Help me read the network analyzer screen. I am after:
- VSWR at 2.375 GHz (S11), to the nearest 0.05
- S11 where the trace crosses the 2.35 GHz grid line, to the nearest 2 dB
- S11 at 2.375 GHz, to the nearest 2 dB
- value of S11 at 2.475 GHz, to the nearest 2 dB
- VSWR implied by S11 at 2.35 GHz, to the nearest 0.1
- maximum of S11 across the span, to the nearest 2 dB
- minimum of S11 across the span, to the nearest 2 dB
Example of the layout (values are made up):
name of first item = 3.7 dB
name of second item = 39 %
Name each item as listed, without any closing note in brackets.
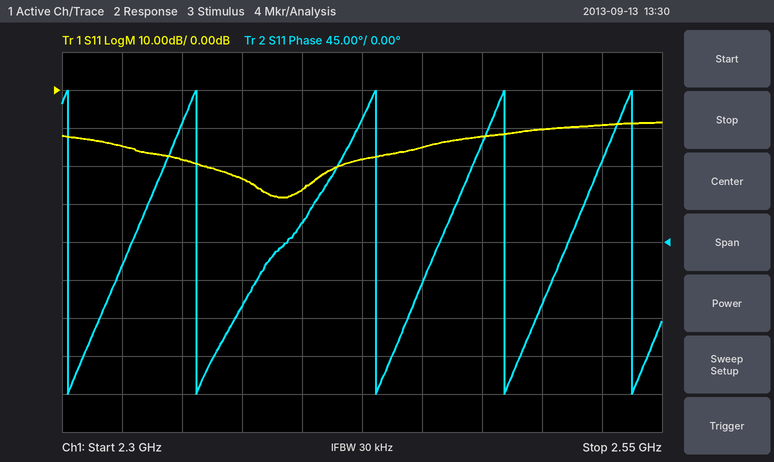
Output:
VSWR at 2.375 GHz (S11), to the nearest 0.05 = 1.15
S11 where the trace crosses the 2.35 GHz grid line, to the nearest 2 dB = -18 dB
S11 at 2.375 GHz, to the nearest 2 dB = -24 dB
value of S11 at 2.475 GHz, to the nearest 2 dB = -12 dB
VSWR implied by S11 at 2.35 GHz, to the nearest 0.1 = 1.3
maximum of S11 across the span, to the nearest 2 dB = -8 dB
minimum of S11 across the span, to the nearest 2 dB = -28 dB
